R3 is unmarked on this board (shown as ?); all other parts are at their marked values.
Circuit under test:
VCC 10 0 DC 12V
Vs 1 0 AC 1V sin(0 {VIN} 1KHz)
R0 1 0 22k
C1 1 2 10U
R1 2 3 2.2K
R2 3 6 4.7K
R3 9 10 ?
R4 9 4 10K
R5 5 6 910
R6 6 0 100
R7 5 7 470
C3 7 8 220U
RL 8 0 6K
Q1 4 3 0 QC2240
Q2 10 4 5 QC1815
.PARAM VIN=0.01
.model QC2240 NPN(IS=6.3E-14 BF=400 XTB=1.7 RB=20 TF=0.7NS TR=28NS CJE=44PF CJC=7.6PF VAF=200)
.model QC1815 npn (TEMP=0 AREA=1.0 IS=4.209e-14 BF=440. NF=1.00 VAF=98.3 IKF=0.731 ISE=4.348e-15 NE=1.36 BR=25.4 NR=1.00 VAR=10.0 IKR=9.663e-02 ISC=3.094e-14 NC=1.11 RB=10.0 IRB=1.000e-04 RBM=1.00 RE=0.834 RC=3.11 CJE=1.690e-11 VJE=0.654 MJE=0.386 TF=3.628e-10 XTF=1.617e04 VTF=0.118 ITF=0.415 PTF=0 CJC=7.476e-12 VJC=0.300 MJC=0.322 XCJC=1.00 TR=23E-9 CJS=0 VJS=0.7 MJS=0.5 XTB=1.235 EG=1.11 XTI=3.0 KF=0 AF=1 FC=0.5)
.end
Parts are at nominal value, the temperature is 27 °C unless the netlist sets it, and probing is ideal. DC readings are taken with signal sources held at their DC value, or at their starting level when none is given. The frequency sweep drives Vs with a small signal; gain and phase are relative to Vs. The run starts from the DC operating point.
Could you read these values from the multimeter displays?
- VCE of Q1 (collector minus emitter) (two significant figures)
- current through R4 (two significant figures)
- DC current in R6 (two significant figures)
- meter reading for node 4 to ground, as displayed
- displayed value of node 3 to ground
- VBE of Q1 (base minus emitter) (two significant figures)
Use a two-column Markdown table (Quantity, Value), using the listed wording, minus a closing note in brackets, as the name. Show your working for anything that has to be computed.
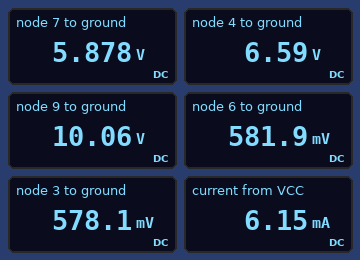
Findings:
| Quantity | Value |
|---|---|
| VCE of Q1 (collector minus emitter) | 6.59 V = 6.6 V |
| current through R4 | (10.06 V - 6.59 V) / 10 kΩ = 350 µA |
| DC current in R6 | (581.9 mV) / 100 Ω = 5.8 mA |
| meter reading for node 4 to ground, as displayed | 6.59 V |
| displayed value of node 3 to ground | 578.1 mV |
| VBE of Q1 (base minus emitter) | 578.1 mV = 580 mV |
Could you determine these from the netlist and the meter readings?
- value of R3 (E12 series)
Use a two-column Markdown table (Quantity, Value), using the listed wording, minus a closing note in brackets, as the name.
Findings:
| Quantity | Value |
|---|---|
| value of R3 | 5.6 kΩ |
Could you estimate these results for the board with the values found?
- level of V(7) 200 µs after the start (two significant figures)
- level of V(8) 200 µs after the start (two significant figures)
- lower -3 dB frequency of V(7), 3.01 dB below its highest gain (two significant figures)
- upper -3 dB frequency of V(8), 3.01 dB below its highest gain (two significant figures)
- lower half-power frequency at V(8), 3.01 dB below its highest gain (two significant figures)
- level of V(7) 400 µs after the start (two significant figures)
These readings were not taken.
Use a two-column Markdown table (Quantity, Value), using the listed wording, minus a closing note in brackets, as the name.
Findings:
| Quantity | Value |
|---|---|
| level of V(7) 200 µs after the start | 5.7 V |
| level of V(8) 200 µs after the start | -160 mV |
| lower -3 dB frequency of V(7), 3.01 dB below its highest gain | 6.5 Hz |
| upper -3 dB frequency of V(8), 3.01 dB below its highest gain | 900 kHz |
| lower half-power frequency at V(8), 3.01 dB below its highest gain | 6.5 Hz |
| level of V(7) 400 µs after the start | 5.8 V |
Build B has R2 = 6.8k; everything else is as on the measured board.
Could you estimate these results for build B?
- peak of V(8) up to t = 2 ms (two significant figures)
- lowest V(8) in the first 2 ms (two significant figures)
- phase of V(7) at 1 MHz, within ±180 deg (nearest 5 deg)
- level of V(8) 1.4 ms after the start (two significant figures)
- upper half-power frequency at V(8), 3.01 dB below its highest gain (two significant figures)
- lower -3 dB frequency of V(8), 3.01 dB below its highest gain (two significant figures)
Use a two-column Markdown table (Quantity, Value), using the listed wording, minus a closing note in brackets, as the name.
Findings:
| Quantity | Value |
|---|---|
| peak of V(8) up to t = 2 ms | 240 mV |
| lowest V(8) in the first 2 ms | -240 mV |
| phase of V(7) at 1 MHz, within ±180 deg | 120 deg |
| level of V(8) 1.4 ms after the start | -140 mV |
| upper half-power frequency at V(8), 3.01 dB below its highest gain | 650 kHz |
| lower -3 dB frequency of V(8), 3.01 dB below its highest gain | 6.2 Hz |
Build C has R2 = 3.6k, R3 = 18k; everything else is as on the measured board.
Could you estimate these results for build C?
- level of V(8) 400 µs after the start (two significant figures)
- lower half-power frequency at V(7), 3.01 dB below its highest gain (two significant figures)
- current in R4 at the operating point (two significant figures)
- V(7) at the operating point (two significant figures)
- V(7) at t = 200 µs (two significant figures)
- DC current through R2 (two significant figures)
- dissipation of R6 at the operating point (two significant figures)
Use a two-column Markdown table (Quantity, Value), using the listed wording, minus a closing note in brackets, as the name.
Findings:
| Quantity | Value |
|---|---|
| level of V(8) 400 µs after the start | -78 mV |
| lower half-power frequency at V(7), 3.01 dB below its highest gain | 6.6 Hz |
| current in R4 at the operating point | 200 µA |
| V(7) at the operating point | 5.7 V |
| V(7) at t = 200 µs | 5.6 V |
| DC current through R2 | 450 nA |
| dissipation of R6 at the operating point | 3.2 mW |
